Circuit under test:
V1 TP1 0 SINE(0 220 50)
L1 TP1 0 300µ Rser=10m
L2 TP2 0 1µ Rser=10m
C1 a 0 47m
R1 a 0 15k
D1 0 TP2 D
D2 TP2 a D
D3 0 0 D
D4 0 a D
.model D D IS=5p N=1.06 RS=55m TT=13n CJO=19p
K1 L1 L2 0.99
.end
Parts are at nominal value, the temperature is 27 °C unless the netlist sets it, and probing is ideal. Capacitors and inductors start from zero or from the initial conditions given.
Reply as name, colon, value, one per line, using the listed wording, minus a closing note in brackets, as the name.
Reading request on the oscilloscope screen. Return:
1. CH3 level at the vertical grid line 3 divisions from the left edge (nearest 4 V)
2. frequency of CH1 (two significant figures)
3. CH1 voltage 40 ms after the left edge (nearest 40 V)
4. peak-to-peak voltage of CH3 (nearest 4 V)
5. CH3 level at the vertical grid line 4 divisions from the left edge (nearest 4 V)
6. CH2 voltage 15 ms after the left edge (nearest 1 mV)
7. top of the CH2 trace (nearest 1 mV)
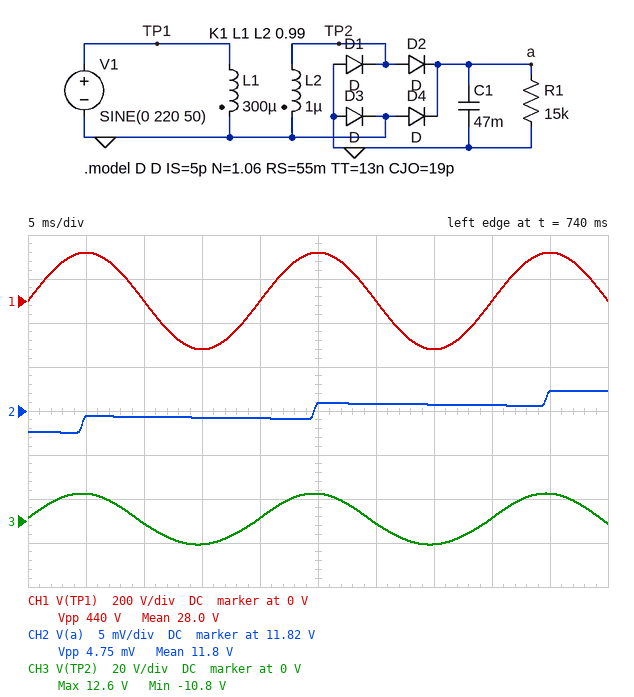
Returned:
CH3 level at the vertical grid line 3 divisions from the left edge: -12 V
frequency of CH1: 50 Hz
CH1 voltage 40 ms after the left edge: 0 V
peak-to-peak voltage of CH3: 24 V
CH3 level at the vertical grid line 4 divisions from the left edge: 0 V
CH2 voltage 15 ms after the left edge: 11.819 V
top of the CH2 trace: 11.822 V
